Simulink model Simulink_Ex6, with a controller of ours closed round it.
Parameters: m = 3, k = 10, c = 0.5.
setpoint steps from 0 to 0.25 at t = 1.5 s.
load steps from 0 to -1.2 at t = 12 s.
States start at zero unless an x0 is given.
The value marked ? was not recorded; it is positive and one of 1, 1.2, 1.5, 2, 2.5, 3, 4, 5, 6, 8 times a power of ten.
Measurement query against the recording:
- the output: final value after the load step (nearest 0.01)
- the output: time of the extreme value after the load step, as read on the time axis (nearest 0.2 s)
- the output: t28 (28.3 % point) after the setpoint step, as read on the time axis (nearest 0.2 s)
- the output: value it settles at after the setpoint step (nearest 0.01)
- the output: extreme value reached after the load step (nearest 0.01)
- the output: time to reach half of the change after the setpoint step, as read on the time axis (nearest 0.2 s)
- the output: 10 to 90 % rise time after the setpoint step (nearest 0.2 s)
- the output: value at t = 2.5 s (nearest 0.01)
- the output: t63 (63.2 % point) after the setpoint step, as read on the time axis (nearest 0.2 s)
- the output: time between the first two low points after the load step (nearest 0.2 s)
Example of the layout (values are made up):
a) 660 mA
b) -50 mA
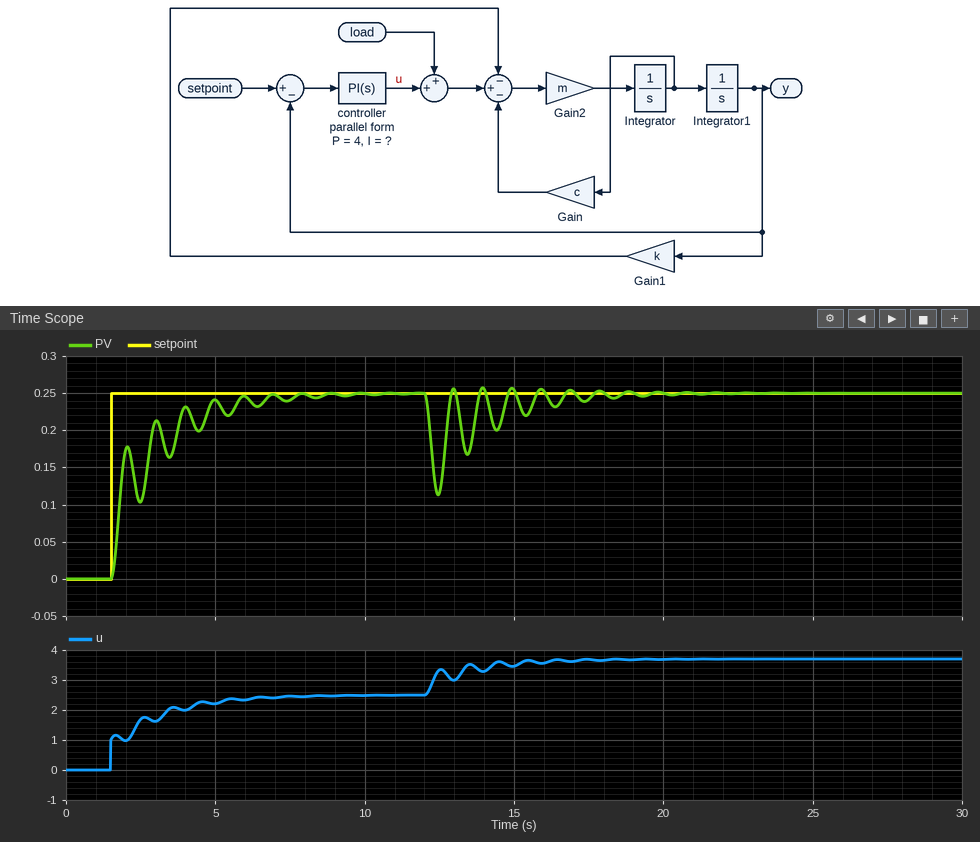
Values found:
a) 0.25
b) 12.4 s
c) 1.8 s
d) 0.25
e) 0.11
f) 1.8 s
g) 2.2 s
h) 0.10
i) 2.0 s
j) 1.0 s
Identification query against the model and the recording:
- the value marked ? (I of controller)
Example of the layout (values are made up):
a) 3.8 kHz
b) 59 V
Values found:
a) 8
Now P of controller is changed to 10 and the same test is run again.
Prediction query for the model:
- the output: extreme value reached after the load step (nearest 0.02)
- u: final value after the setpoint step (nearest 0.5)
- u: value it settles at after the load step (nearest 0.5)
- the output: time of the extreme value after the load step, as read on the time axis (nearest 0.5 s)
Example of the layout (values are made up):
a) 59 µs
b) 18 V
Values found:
a) 0.14
b) 2.5
c) 3.5
d) 12.5 s
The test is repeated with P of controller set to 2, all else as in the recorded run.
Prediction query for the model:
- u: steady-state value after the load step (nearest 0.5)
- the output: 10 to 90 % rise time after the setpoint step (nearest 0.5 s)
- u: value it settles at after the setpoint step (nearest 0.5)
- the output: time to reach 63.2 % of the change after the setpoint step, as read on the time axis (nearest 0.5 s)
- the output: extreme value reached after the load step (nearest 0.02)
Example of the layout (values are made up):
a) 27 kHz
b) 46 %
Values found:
a) 3.5
b) 2.5 s
c) 2.5
d) 3.0 s
e) 0.10
